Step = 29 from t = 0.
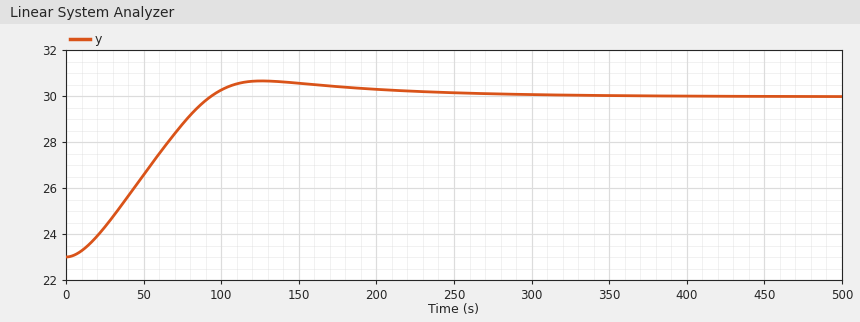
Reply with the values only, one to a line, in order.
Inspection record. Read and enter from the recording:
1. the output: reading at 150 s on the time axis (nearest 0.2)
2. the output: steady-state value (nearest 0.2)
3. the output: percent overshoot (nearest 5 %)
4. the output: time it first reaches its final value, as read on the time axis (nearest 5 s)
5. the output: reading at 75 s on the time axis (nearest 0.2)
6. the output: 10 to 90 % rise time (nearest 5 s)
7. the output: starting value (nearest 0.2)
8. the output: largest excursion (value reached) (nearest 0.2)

30.6
30.0
10 %
95 s
28.8
65 s
23.0
30.6
